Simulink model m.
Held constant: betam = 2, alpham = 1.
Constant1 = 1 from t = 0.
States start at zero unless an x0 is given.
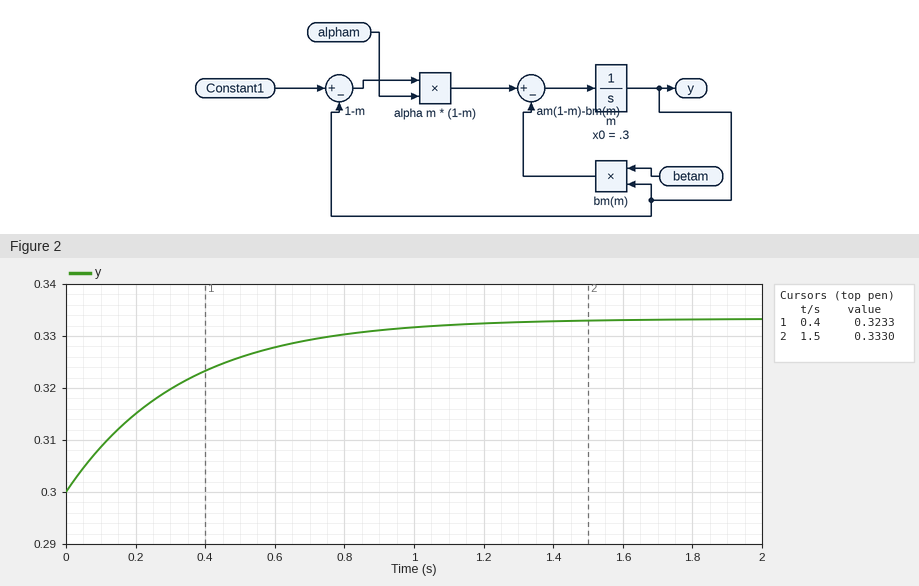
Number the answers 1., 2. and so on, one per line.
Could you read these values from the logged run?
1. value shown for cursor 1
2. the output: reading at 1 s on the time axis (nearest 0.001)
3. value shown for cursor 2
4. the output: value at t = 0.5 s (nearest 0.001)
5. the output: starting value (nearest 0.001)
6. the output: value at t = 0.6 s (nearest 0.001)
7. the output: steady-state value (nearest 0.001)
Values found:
1. 0.3233
2. 0.332
3. 0.3330
4. 0.326
5. 0.300
6. 0.328
7. 0.333
